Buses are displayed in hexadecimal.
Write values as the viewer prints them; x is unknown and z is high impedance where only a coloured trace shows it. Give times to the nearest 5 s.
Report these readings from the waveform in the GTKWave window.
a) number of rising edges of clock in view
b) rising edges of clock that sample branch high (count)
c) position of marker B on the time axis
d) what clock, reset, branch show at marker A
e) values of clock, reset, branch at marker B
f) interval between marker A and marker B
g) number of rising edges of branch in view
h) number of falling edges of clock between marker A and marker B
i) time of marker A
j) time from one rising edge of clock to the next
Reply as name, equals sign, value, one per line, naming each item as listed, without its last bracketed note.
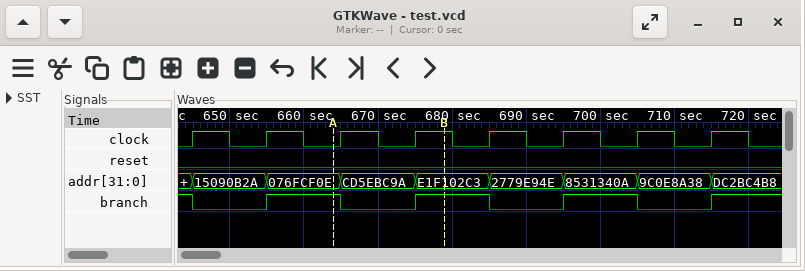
number of rising edges of clock in view = 8
rising edges of clock that sample branch high = 4
position of marker B on the time axis = 680 s
what clock, reset, branch show at marker A = clock=0, reset=0, branch=1
values of clock, reset, branch at marker B = clock=1, reset=0, branch=1
interval between marker A and marker B = 15 s
number of rising edges of branch in view = 4
number of falling edges of clock between marker A and marker B = 1
time of marker A = 665 s
time from one rising edge of clock to the next = 10 s
